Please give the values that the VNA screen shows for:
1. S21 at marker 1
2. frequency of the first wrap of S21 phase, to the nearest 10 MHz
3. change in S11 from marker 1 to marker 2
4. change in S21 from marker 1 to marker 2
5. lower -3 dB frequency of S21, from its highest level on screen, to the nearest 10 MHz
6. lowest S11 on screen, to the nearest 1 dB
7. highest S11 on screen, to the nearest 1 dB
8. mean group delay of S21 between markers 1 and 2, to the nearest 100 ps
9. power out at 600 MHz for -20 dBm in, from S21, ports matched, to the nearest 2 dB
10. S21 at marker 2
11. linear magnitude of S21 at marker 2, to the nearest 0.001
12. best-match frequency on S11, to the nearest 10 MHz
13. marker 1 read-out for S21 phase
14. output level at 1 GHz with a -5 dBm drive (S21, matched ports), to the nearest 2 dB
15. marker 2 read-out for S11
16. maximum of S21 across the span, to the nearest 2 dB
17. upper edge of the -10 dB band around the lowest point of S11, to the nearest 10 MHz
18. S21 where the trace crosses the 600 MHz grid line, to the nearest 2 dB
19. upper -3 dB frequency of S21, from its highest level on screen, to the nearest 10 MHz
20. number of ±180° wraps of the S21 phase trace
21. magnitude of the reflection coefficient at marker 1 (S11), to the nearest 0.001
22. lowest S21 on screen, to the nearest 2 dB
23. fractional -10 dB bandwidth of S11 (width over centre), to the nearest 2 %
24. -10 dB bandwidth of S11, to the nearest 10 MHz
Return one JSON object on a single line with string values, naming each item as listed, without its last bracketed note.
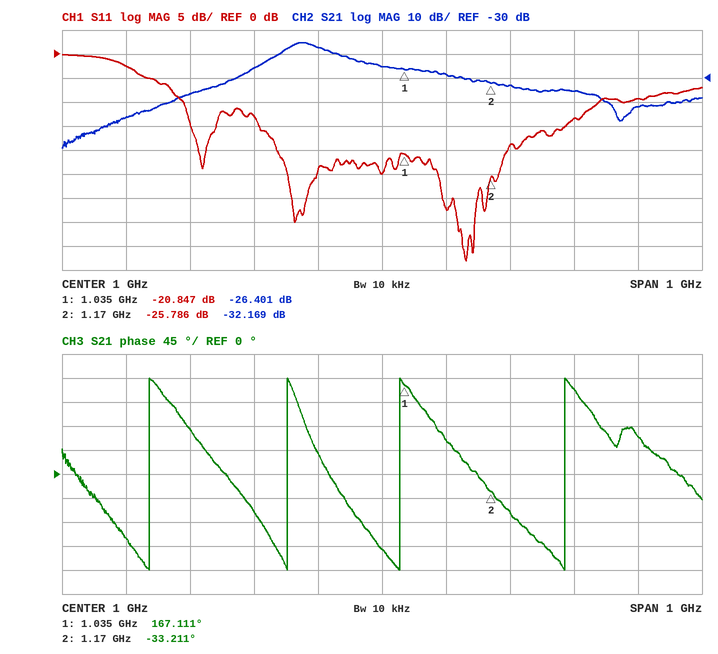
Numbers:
{"S21 at marker 1": "-26.401 dB", "frequency of the first wrap of S21 phase, to the nearest 10 MHz": "640 MHz", "change in S11 from marker 1 to marker 2": "-4.939 dB", "change in S21 from marker 1 to marker 2": "-5.768 dB", "lower -3 dB frequency of S21, from its highest level on screen, to the nearest 10 MHz": "850 MHz", "lowest S11 on screen, to the nearest 1 dB": "-43 dB", "highest S11 on screen, to the nearest 1 dB": "0 dB", "mean group delay of S21 between markers 1 and 2, to the nearest 100 ps": "4.1 ns", "power out at 600 MHz for -20 dBm in, from S21, ports matched, to the nearest 2 dB": "-66 dBm", "S21 at marker 2": "-32.169 dB", "linear magnitude of S21 at marker 2, to the nearest 0.001": "0.025", "best-match frequency on S11, to the nearest 10 MHz": "1.13 GHz", "marker 1 read-out for S21 phase": "167.111°", "output level at 1 GHz with a -5 dBm drive (S21, matched ports), to the nearest 2 dB": "-30 dBm", "marker 2 read-out for S11": "-25.786 dB", "maximum of S21 across the span, to the nearest 2 dB": "-16 dB", "upper edge of the -10 dB band around the lowest point of S11, to the nearest 10 MHz": "1.34 GHz", "S21 where the trace crosses the 600 MHz grid line, to the nearest 2 dB": "-46 dB", "upper -3 dB frequency of S21, from its highest level on screen, to the nearest 10 MHz": "910 MHz", "number of ±180° wraps of the S21 phase trace": "4", "magnitude of the reflection coefficient at marker 1 (S11), to the nearest 0.001": "0.091", "lowest S21 on screen, to the nearest 2 dB": "-60 dB", "fractional -10 dB bandwidth of S11 (width over centre), to the nearest 2 %": "64 %", "-10 dB bandwidth of S11, to the nearest 10 MHz": "650 MHz"}
